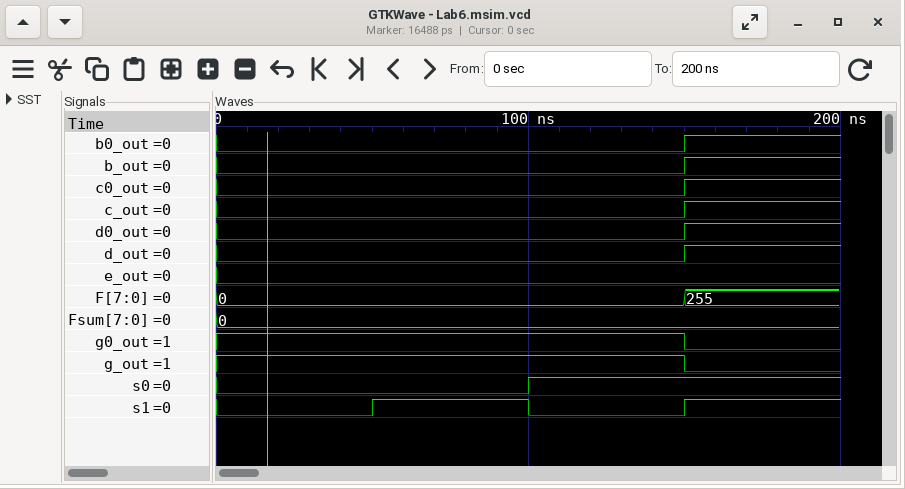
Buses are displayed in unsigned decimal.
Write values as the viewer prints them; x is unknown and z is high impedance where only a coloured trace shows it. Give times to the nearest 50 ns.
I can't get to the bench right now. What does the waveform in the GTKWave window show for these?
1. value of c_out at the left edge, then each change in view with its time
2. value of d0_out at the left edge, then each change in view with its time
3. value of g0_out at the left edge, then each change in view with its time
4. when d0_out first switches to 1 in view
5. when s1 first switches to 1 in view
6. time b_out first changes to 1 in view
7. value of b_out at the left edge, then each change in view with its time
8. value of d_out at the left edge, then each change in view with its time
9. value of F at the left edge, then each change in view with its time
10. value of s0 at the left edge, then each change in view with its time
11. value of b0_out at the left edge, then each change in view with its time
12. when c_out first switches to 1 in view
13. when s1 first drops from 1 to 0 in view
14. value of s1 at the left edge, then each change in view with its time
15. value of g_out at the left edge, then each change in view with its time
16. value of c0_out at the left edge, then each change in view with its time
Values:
0, 1 at 150 ns
0, 1 at 150 ns
1, 0 at 150 ns
150 ns
50 ns
150 ns
0, 1 at 150 ns
0, 1 at 150 ns
0, 255 at 150 ns
0, 1 at 100 ns
0, 1 at 150 ns
150 ns
100 ns
0, 1 at 50 ns, 0 at 100 ns, 1 at 150 ns
1, 0 at 150 ns
0, 1 at 150 ns
